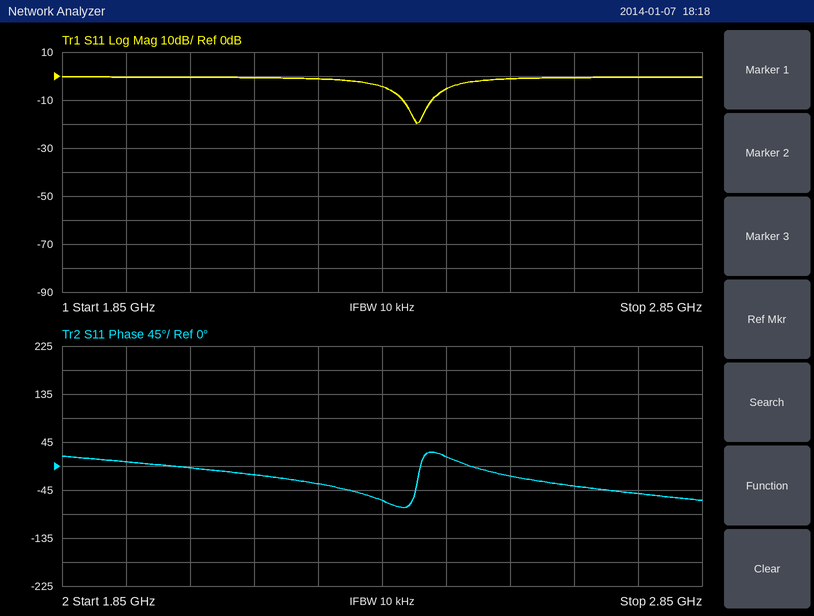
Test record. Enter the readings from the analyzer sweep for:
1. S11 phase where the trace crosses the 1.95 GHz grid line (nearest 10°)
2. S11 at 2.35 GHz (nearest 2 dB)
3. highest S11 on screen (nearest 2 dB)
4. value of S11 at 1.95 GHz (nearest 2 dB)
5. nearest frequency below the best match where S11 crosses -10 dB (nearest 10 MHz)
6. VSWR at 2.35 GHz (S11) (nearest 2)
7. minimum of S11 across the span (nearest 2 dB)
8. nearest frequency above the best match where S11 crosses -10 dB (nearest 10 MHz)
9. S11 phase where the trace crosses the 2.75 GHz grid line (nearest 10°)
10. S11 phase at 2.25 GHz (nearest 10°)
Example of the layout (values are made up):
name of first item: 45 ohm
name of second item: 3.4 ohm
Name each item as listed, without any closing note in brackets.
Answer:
S11 phase where the trace crosses the 1.95 GHz grid line: 10°
S11 at 2.35 GHz: -4 dB
highest S11 on screen: 0 dB
value of S11 at 1.95 GHz: 0 dB
nearest frequency below the best match where S11 crosses -10 dB: 2.38 GHz
VSWR at 2.35 GHz (S11): 4
minimum of S11 across the span: -20 dB
nearest frequency above the best match where S11 crosses -10 dB: 2.43 GHz
S11 phase where the trace crosses the 2.75 GHz grid line: -50°
S11 phase at 2.25 GHz: -30°
